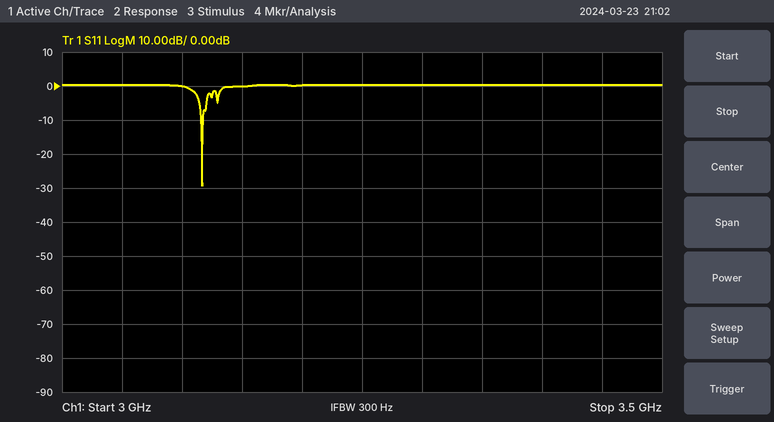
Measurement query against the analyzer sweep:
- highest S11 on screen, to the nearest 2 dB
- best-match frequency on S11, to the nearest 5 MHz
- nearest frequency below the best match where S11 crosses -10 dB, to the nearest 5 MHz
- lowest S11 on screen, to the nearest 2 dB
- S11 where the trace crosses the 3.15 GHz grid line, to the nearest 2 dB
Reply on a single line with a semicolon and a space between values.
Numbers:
0 dB; 3.115 GHz; 3.115 GHz; -30 dB; 0 dB
